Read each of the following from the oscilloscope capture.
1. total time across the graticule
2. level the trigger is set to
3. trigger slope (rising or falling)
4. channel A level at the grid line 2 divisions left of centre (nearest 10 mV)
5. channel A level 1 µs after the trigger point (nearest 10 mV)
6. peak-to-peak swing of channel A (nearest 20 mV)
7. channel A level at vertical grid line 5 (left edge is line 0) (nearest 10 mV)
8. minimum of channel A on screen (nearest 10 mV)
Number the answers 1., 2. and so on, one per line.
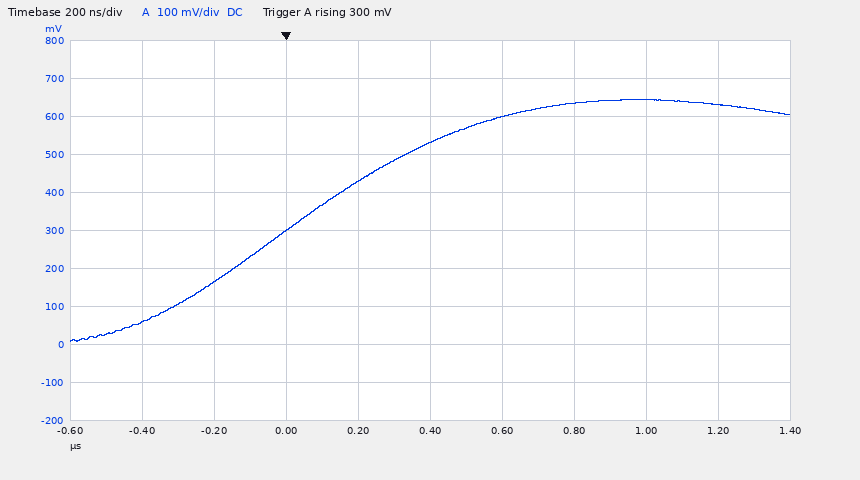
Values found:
1. 2 µs
2. 300 mV
3. rising
4. 300 mV
5. 640 mV
6. 640 mV
7. 530 mV
8. 10 mV
